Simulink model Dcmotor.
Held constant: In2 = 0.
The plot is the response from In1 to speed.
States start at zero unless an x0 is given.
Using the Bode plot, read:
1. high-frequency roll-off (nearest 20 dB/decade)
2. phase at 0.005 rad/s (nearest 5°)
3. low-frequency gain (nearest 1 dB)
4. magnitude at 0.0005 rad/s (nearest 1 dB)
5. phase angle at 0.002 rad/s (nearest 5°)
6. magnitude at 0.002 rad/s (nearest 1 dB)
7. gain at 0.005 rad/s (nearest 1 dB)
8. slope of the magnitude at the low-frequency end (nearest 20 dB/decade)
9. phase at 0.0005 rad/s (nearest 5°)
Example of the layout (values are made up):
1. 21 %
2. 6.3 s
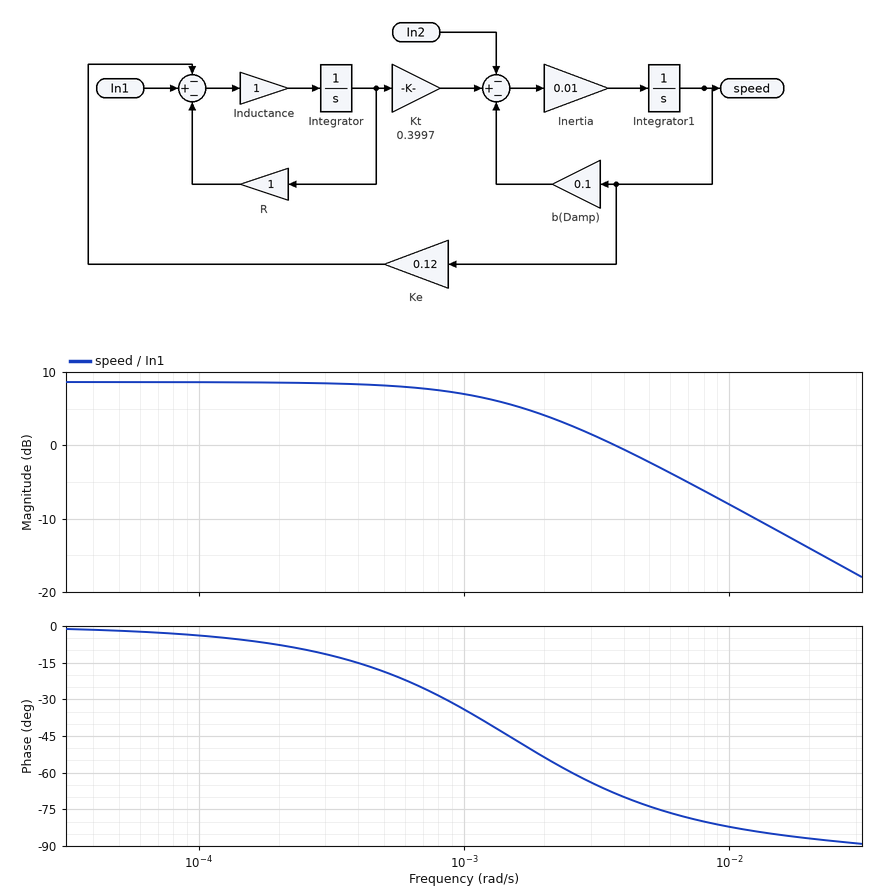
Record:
1. -20 dB/decade
2. -75°
3. 9 dB
4. 8 dB
5. -55°
6. 4 dB
7. -2 dB
8. 0 dB/decade
9. -20°
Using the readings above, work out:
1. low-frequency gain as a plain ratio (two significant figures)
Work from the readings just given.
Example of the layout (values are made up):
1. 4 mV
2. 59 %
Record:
1. 2.8
